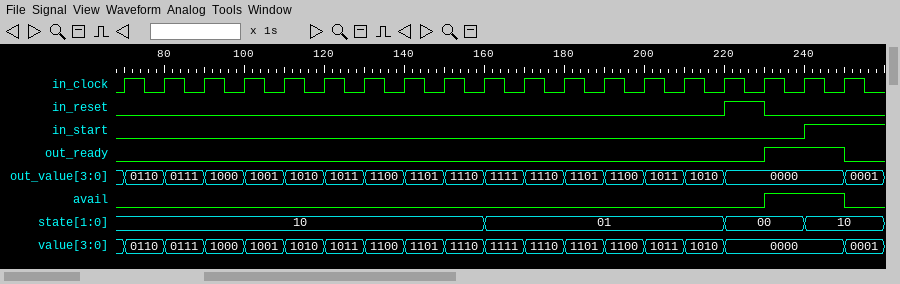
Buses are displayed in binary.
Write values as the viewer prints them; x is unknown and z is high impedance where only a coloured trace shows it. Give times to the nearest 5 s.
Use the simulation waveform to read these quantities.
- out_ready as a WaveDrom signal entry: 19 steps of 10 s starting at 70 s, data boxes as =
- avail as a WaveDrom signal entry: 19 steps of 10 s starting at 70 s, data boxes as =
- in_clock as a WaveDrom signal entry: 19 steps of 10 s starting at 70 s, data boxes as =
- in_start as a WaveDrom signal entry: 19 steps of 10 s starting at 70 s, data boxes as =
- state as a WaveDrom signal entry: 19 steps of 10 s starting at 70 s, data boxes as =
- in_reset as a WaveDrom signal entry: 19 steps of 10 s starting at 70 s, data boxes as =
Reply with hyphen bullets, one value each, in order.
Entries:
- {name: 'out_ready', wave: '0...............1.0'}
- {name: 'avail', wave: '0...............1.0'}
- {name: 'in_clock', wave: 'p..................'}
- {name: 'in_start', wave: '0................1.'}
- {name: 'state', wave: '=........=.....=.=.', data: '10 01 00 10'}
- {name: 'in_reset', wave: '0..............10..'}
